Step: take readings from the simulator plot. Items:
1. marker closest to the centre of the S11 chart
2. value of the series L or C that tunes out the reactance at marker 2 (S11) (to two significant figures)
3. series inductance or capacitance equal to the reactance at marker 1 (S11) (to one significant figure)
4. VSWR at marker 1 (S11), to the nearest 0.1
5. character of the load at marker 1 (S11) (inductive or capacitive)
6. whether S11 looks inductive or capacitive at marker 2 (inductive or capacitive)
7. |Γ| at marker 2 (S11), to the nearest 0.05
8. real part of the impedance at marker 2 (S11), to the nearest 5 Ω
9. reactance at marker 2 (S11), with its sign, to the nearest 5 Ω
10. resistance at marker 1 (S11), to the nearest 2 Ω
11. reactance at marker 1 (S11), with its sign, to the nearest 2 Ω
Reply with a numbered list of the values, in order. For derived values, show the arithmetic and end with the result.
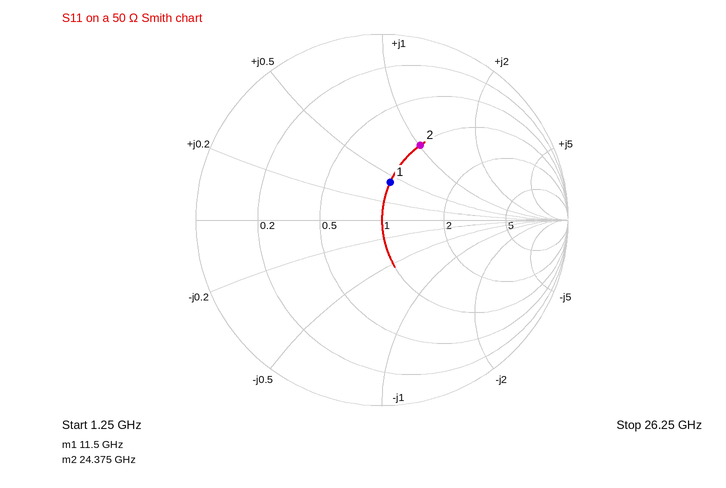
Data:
1. marker 1
2. C = 1/(2π × 24.375 GHz × 50 Ω) ≈ 131 fF, so 130 fF to two significant figures
3. L = 22 Ω/(2π × 11.5 GHz) ≈ 304 pH, so 300 pH to one significant figure
4. 1.5
5. inductive
6. inductive
7. 0.45
8. 50 Ω
9. +50 Ω
10. 50 Ω
11. +22 Ω
